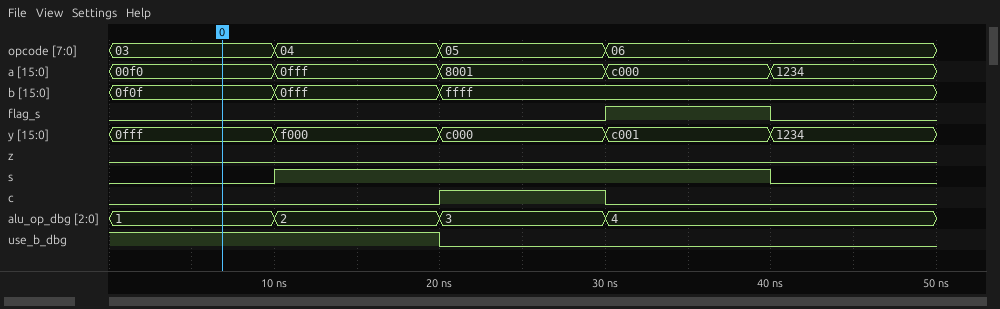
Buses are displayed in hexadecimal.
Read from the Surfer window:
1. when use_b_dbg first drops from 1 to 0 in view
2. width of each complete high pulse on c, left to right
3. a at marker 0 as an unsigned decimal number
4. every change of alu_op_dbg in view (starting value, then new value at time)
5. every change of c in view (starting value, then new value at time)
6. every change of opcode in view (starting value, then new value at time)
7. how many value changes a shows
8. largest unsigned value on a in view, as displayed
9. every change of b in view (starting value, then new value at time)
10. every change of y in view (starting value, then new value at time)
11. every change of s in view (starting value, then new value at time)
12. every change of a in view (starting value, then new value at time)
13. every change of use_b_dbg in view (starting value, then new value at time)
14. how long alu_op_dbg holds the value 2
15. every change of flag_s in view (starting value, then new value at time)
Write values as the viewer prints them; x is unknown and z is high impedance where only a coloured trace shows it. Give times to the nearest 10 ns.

20 ns
10 ns
240
1, 2 at 10 ns, 3 at 20 ns, 4 at 30 ns
0, 1 at 20 ns, 0 at 30 ns
03, 04 at 10 ns, 05 at 20 ns, 06 at 30 ns
4
c000
0f0f, 0fff at 10 ns, ffff at 20 ns
0fff, f000 at 10 ns, c000 at 20 ns, c001 at 30 ns, 1234 at 40 ns
0, 1 at 10 ns, 0 at 40 ns
00f0, 0fff at 10 ns, 8001 at 20 ns, c000 at 30 ns, 1234 at 40 ns
1, 0 at 20 ns
10 ns
0, 1 at 30 ns, 0 at 40 ns
